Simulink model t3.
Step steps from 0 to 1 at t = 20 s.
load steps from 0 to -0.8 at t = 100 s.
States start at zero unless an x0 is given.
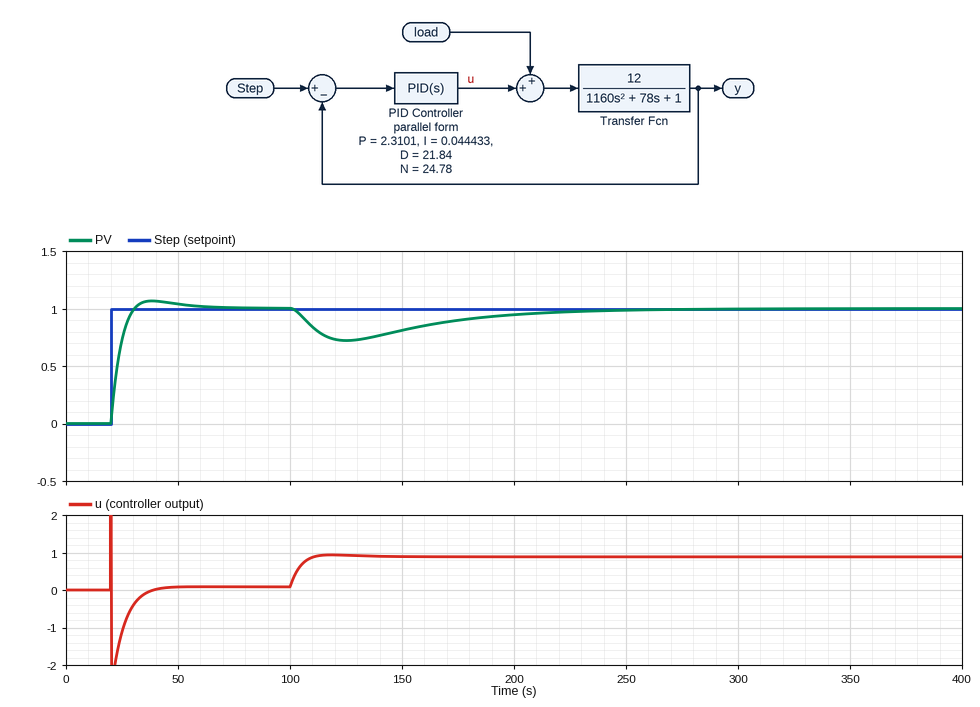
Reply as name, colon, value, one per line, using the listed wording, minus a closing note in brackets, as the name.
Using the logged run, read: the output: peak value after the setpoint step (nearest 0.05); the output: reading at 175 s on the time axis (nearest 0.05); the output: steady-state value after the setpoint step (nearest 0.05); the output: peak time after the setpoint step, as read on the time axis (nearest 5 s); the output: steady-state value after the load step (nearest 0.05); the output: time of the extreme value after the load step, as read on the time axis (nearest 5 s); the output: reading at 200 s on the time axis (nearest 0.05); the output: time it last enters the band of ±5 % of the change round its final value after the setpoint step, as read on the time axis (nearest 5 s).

the output: peak value after the setpoint step: 1.05
the output: reading at 175 s on the time axis: 0.90
the output: steady-state value after the setpoint step: 1.00
the output: peak time after the setpoint step, as read on the time axis: 40 s
the output: steady-state value after the load step: 1.00
the output: time of the extreme value after the load step, as read on the time axis: 125 s
the output: reading at 200 s on the time axis: 0.95
the output: time it last enters the band of ±5 % of the change round its final value after the setpoint step, as read on the time axis: 45 s
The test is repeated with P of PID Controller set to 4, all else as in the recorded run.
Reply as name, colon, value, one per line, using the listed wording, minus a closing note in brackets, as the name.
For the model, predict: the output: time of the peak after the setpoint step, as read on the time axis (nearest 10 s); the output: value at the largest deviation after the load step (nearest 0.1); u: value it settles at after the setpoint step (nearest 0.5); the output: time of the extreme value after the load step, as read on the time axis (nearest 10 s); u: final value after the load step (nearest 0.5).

the output: time of the peak after the setpoint step, as read on the time axis: 30 s
the output: value at the largest deviation after the load step: 0.8
u: value it settles at after the setpoint step: 0.0
the output: time of the extreme value after the load step, as read on the time axis: 120 s
u: final value after the load step: 1.0
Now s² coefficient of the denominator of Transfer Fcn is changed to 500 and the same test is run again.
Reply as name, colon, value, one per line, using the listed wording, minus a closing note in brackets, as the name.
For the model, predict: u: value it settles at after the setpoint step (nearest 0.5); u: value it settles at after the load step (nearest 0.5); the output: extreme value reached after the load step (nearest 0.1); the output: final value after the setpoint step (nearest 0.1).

u: value it settles at after the setpoint step: 0.0
u: value it settles at after the load step: 1.0
the output: extreme value reached after the load step: 0.7
the output: final value after the setpoint step: 1.0
